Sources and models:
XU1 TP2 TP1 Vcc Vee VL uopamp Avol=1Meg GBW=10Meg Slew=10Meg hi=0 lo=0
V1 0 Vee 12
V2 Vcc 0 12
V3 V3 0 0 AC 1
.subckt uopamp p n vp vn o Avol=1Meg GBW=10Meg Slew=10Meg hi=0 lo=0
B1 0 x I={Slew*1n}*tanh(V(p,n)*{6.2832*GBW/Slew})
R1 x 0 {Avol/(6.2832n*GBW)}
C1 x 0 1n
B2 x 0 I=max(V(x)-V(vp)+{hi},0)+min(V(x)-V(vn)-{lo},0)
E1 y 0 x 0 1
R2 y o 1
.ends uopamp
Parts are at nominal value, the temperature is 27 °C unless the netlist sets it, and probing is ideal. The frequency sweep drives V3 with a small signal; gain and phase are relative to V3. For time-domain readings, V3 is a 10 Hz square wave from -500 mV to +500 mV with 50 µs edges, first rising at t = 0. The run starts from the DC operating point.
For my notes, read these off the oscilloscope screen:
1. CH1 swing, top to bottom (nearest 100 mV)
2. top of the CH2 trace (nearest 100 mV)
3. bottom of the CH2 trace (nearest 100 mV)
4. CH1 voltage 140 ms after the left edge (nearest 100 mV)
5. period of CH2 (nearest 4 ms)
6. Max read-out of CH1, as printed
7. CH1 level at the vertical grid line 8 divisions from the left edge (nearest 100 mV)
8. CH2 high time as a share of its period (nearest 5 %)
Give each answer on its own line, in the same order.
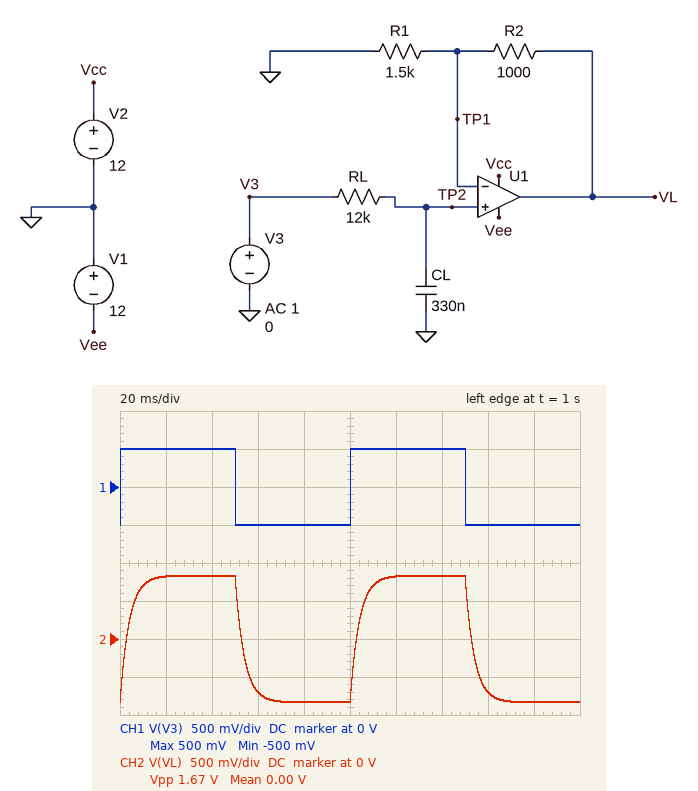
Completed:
1.0 V
800 mV
-800 mV
500 mV
100 ms
500 mV
-500 mV
50 %
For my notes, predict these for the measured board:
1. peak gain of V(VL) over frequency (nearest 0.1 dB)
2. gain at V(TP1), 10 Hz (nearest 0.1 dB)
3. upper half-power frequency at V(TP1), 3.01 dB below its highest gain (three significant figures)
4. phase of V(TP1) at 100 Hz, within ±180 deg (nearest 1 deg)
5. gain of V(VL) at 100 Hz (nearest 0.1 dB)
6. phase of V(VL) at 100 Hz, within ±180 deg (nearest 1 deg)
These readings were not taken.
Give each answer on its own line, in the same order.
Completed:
4.4 dB
-0.3 dB
40.2 Hz
-68 deg
-4.1 dB
-68 deg
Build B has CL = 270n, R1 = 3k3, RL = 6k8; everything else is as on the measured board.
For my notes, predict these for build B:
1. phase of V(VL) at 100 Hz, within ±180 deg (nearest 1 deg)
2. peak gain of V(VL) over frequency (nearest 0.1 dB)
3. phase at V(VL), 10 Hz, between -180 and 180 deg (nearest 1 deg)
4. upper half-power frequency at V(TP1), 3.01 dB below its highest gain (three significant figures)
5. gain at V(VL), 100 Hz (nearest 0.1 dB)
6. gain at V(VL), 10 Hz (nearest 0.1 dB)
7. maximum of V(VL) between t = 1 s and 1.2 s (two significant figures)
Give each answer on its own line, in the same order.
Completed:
-49 deg
2.3 dB
-7 deg
86.7 Hz
-1.4 dB
2.2 dB
650 mV
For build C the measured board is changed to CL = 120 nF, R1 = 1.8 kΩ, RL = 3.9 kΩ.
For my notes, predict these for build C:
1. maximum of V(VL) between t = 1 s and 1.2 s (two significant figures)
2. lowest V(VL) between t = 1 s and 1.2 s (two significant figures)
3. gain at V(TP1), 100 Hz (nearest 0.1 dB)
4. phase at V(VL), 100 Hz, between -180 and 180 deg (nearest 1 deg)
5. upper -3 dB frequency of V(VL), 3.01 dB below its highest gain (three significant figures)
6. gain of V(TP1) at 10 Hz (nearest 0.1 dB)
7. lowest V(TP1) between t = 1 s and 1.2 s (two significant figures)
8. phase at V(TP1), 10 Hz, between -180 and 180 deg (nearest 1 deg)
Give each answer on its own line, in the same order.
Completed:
780 mV
-780 mV
-0.4 dB
-16 deg
340 Hz
0 dB
-500 mV
-2 deg
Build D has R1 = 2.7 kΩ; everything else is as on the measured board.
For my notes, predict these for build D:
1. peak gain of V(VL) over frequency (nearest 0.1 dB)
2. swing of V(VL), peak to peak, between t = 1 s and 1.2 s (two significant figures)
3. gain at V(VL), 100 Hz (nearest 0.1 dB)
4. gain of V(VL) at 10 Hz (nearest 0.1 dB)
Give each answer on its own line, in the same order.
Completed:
2.7 dB
1.4 V
-5.8 dB
2.5 dB
